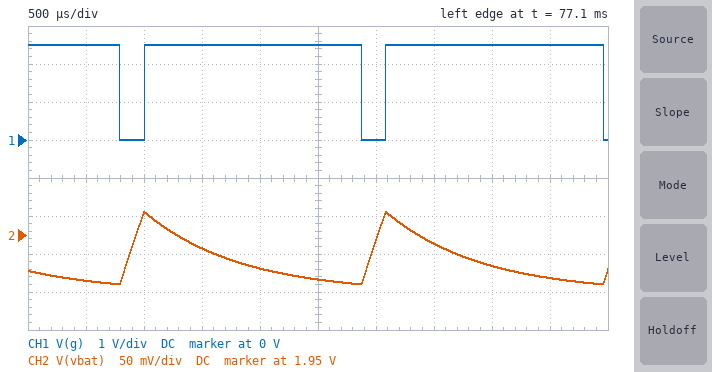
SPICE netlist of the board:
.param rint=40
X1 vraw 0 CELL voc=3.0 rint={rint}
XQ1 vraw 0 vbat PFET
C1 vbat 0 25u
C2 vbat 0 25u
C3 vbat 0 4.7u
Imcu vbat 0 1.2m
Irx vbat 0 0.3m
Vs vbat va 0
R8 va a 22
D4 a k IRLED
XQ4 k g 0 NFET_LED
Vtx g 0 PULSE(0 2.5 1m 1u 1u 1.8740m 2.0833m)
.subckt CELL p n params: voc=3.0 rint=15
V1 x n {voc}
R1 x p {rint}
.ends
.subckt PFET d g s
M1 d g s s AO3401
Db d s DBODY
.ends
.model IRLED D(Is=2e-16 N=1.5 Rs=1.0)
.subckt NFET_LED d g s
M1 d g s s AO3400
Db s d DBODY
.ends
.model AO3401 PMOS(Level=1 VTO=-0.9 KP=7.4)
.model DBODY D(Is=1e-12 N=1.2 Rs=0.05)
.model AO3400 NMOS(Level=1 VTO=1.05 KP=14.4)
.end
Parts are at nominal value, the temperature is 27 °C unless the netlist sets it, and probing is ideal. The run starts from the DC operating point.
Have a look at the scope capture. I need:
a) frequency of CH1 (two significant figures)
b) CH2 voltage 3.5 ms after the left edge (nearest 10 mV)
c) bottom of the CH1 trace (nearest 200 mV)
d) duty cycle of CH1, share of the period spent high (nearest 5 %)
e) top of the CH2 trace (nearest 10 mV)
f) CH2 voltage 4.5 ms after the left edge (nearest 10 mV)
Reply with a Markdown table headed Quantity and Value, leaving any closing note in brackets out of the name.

| Quantity | Value |
|---|---|
| frequency of CH1 | 480 Hz |
| CH2 voltage 3.5 ms after the left edge | 1.94 V |
| bottom of the CH1 trace | 0 V |
| duty cycle of CH1, share of the period spent high | 90 % |
| top of the CH2 trace | 1.98 V |
| CH2 voltage 4.5 ms after the left edge | 1.89 V |
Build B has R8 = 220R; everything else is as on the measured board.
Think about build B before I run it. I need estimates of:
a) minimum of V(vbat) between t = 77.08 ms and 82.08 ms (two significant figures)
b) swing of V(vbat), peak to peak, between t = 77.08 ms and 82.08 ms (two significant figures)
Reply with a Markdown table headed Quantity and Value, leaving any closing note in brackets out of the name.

| Quantity | Value |
|---|---|
| minimum of V(vbat) between t = 77.08 ms and 82.08 ms | 2.7 V |
| swing of V(vbat), peak to peak, between t = 77.08 ms and 82.08 ms | 23 mV |
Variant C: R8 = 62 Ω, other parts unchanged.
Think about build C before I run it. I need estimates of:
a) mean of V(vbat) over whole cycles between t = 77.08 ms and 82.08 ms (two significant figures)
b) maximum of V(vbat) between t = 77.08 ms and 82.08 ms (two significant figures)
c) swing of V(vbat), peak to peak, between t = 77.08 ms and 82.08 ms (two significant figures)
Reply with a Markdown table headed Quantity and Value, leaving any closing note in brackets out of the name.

| Quantity | Value |
|---|---|
| mean of V(vbat) over whole cycles between t = 77.08 ms and 82.08 ms | 2.3 V |
| maximum of V(vbat) between t = 77.08 ms and 82.08 ms | 2.4 V |
| swing of V(vbat), peak to peak, between t = 77.08 ms and 82.08 ms | 58 mV |
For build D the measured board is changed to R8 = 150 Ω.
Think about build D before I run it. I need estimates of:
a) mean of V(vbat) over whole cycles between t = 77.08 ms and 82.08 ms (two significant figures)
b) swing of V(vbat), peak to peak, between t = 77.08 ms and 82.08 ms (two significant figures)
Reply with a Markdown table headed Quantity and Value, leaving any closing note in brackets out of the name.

| Quantity | Value |
|---|---|
| mean of V(vbat) over whole cycles between t = 77.08 ms and 82.08 ms | 2.6 V |
| swing of V(vbat), peak to peak, between t = 77.08 ms and 82.08 ms | 31 mV |
